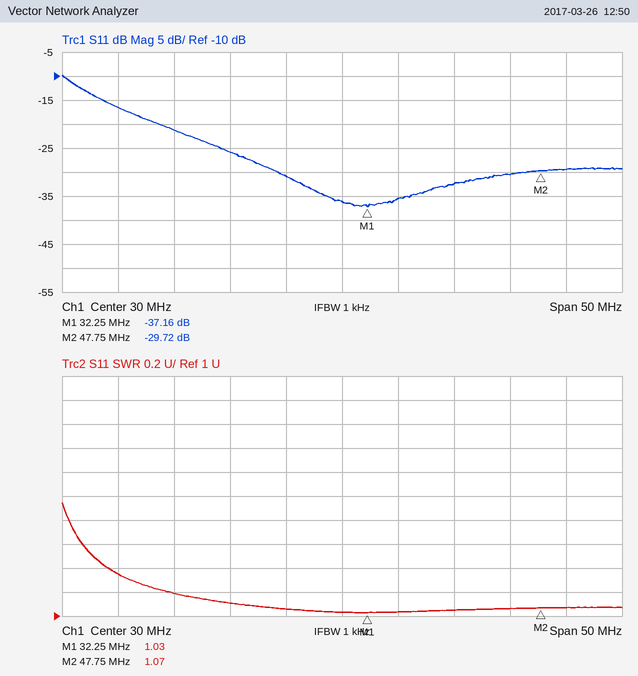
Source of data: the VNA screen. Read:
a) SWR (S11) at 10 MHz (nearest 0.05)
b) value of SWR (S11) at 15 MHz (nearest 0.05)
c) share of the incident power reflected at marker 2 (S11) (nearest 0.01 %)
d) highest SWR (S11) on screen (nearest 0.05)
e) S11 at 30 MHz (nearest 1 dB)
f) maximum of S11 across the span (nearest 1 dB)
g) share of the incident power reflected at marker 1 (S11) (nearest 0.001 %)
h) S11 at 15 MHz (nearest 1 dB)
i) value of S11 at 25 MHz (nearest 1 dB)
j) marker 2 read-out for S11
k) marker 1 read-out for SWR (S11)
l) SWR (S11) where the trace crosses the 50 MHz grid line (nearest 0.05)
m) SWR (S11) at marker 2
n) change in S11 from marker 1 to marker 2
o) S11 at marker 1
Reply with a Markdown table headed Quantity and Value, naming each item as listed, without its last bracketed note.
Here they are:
| Quantity | Value |
|---|---|
| SWR (S11) at 10 MHz | 1.35 |
| value of SWR (S11) at 15 MHz | 1.20 |
| share of the incident power reflected at marker 2 (S11) | 0.11 % |
| highest SWR (S11) on screen | 1.95 |
| S11 at 30 MHz | -36 dB |
| maximum of S11 across the span | -10 dB |
| share of the incident power reflected at marker 1 (S11) | 0.019 % |
| S11 at 15 MHz | -21 dB |
| value of S11 at 25 MHz | -31 dB |
| marker 2 read-out for S11 | -29.72 dB |
| marker 1 read-out for SWR | 1.03 |
| SWR (S11) where the trace crosses the 50 MHz grid line | 1.05 |
| SWR (S11) at marker 2 | 1.07 |
| change in S11 from marker 1 to marker 2 | 7.44 dB |
| S11 at marker 1 | -37.16 dB |
